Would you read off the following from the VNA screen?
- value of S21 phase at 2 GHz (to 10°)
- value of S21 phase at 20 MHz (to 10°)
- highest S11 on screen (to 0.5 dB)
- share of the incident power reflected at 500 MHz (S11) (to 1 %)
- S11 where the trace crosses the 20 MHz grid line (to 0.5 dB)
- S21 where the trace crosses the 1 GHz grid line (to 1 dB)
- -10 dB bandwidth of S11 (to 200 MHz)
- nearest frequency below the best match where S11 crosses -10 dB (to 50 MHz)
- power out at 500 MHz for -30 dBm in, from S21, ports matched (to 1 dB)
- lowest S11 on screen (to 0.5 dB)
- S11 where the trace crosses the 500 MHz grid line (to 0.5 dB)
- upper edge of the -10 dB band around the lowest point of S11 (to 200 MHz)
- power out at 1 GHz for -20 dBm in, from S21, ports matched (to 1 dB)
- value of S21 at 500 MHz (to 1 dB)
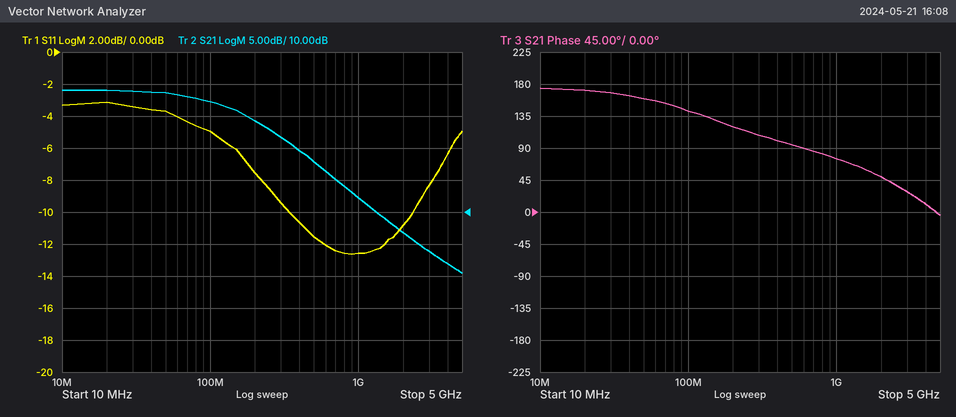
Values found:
50°
170°
-3.0 dB
7 %
-3.0 dB
12 dB
2.0 GHz
350 MHz
-12 dBm
-12.5 dB
-11.5 dB
2.4 GHz
-8 dBm
18 dB
